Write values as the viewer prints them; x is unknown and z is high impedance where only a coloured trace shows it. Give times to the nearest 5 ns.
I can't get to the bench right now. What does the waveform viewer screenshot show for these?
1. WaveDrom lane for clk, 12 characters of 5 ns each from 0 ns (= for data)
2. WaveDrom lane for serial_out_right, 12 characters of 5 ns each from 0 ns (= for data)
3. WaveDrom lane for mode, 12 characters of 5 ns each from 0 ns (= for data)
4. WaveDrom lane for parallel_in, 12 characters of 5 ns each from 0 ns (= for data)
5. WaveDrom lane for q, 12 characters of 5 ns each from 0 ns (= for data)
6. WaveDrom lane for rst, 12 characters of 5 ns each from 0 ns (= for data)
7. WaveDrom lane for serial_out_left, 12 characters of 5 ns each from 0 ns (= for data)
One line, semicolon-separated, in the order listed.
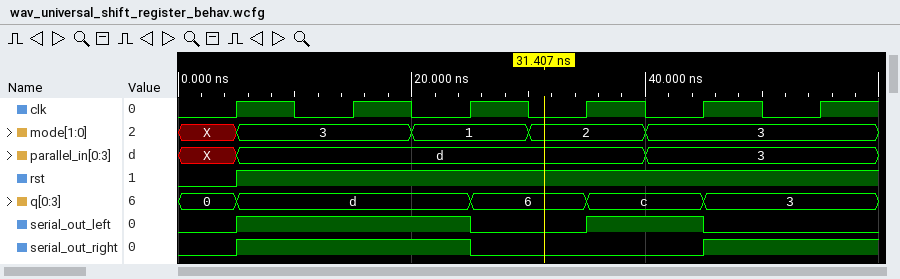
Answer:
{name: 'clk', wave: '010101010101'}; {name: 'serial_out_right', wave: '01...0...1..'}; {name: 'mode', wave: 'x=..=.=.=...', data: '3 1 2 3'}; {name: 'parallel_in', wave: 'x=......=...', data: 'd 3'}; {name: 'q', wave: '==...=.=.=..', data: '0 d 6 c 3'}; {name: 'rst', wave: '01..........'}; {name: 'serial_out_left', wave: '01...0.1.0..'}
